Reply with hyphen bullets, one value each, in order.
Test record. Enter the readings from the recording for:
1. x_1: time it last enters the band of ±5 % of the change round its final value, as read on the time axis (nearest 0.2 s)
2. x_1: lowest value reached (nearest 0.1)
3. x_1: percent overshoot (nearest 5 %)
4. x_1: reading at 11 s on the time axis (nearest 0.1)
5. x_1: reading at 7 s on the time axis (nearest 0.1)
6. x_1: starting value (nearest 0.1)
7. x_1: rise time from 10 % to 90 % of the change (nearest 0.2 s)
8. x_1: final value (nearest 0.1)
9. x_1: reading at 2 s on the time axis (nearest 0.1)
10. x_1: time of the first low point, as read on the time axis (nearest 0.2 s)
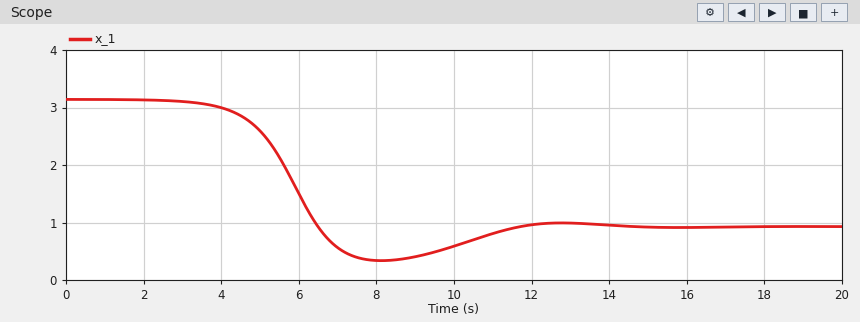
- 11.0 s
- 0.3
- 25 %
- 0.8
- 0.6
- 3.1
- 2.0 s
- 0.9
- 3.1
- 8.2 s
